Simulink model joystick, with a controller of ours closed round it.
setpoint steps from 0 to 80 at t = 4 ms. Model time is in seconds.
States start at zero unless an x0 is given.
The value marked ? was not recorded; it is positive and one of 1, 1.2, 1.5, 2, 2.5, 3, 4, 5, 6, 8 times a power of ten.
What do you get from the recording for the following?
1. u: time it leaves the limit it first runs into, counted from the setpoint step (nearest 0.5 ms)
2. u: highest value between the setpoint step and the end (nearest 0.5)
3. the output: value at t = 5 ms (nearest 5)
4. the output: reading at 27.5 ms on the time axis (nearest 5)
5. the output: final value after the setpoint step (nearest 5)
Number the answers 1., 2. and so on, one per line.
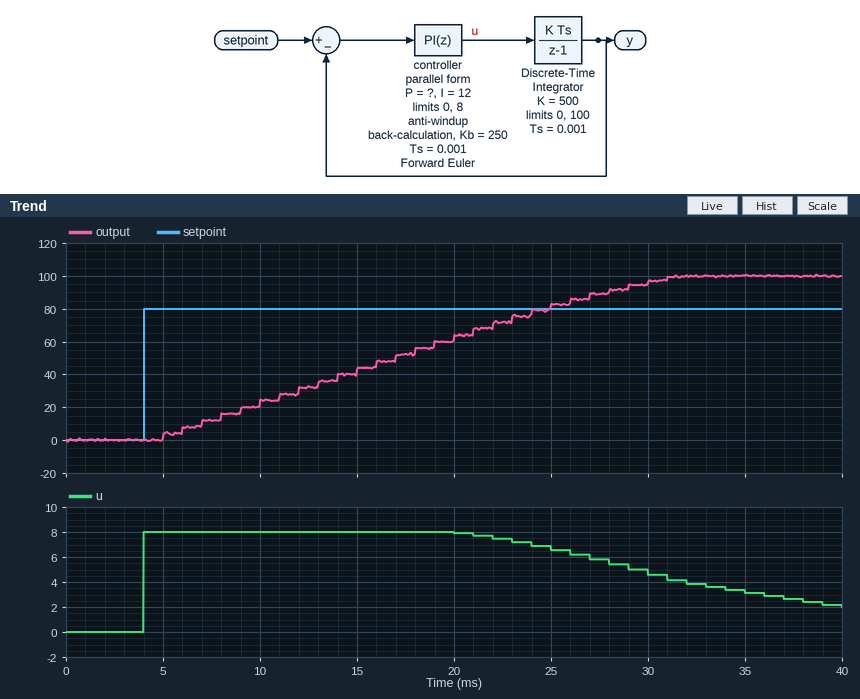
1. 17.0 ms
2. 8.0
3. 5
4. 90
5. 100
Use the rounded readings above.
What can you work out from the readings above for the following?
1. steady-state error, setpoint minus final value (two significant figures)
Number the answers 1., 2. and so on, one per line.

1. -20
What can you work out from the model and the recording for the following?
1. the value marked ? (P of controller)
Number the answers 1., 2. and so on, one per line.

1. 0.1
